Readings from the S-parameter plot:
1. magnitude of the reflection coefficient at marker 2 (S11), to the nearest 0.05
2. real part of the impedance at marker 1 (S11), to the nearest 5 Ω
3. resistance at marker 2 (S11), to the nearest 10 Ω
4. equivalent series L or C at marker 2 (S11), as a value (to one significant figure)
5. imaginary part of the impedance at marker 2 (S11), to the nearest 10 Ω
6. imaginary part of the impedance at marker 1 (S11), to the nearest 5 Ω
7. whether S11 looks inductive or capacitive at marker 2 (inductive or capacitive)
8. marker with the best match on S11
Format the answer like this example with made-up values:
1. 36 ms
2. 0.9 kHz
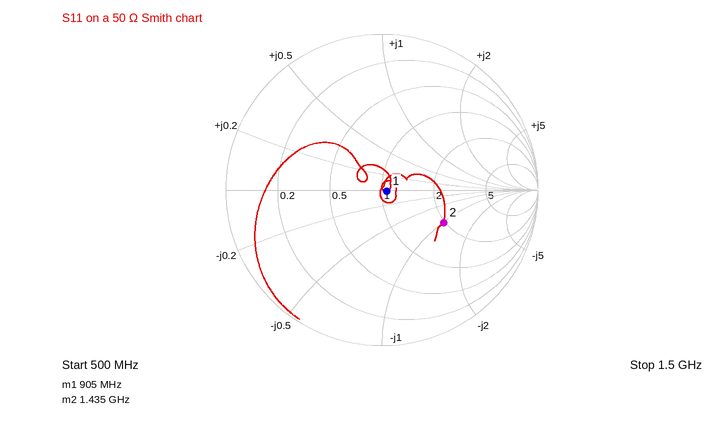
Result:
1. 0.45
2. 55 Ω
3. 100 Ω
4. 2 pF
5. -50 Ω
6. 0 Ω
7. capacitive
8. marker 1
